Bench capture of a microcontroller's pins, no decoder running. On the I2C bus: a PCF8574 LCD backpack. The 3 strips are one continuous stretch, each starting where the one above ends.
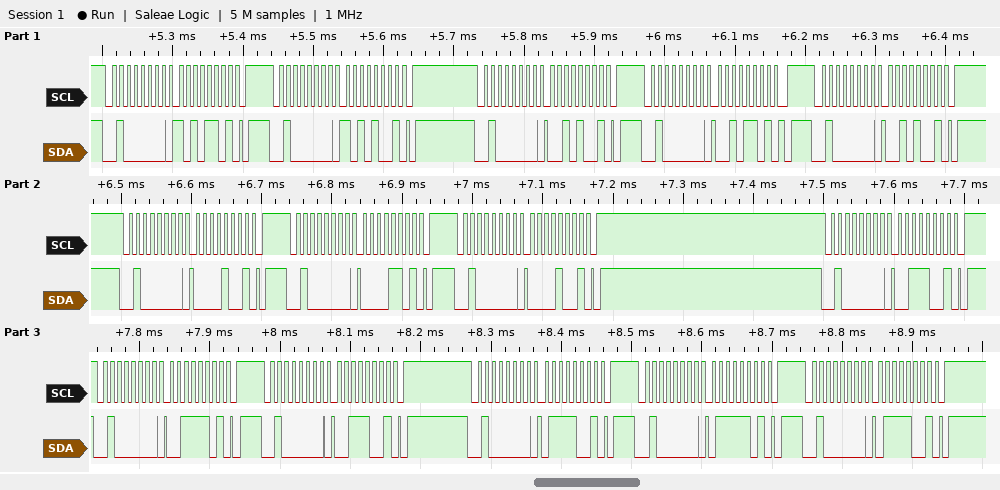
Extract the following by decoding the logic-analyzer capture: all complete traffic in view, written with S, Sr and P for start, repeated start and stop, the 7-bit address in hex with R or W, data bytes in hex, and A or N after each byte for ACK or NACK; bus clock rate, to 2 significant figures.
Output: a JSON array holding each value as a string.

["S 20W A AD A P S 20W A A9 A P S 20W A 29 A P S 20W A 2D A P S 20W A 29 A P S 20W A 09 A P S 20W A 0D A P S 20W A 09 A P S 20W A 39 A P S 20W A 3D A P S 20W A 39 A P S 20W A 79 A P S 20W A 7D A P S 20W A 79 A P", "100 kHz"]
